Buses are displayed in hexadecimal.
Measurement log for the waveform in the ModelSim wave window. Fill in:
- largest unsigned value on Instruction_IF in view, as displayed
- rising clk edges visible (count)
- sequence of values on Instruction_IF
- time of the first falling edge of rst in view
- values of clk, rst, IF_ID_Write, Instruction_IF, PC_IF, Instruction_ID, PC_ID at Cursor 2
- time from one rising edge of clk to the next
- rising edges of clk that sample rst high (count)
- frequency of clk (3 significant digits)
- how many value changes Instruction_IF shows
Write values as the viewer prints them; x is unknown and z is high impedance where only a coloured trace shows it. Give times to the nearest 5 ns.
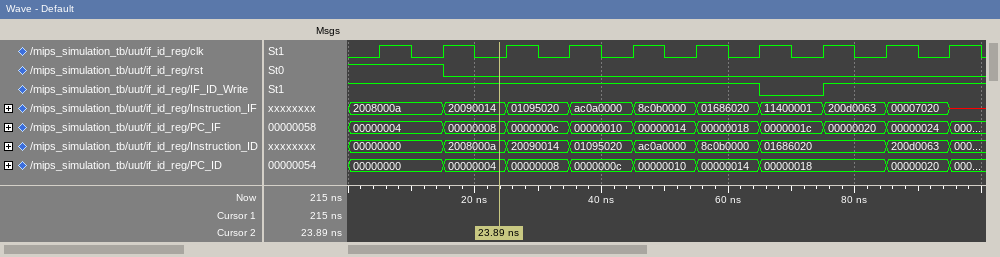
ac0a0000
10
2008000a, 20090014, 01095020, ac0a0000, 8c0b0000, 01686020, 11400001, 200d0063, 00007020, x
15 ns
clk=0, rst=0, IF_ID_Write=1, Instruction_IF=20090014, PC_IF=00000008, Instruction_ID=2008000a, PC_ID=00000004
10 ns
2
100 MHz
9
